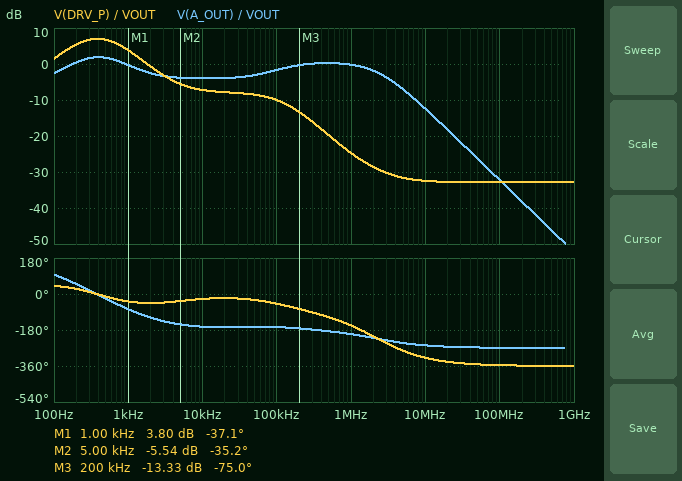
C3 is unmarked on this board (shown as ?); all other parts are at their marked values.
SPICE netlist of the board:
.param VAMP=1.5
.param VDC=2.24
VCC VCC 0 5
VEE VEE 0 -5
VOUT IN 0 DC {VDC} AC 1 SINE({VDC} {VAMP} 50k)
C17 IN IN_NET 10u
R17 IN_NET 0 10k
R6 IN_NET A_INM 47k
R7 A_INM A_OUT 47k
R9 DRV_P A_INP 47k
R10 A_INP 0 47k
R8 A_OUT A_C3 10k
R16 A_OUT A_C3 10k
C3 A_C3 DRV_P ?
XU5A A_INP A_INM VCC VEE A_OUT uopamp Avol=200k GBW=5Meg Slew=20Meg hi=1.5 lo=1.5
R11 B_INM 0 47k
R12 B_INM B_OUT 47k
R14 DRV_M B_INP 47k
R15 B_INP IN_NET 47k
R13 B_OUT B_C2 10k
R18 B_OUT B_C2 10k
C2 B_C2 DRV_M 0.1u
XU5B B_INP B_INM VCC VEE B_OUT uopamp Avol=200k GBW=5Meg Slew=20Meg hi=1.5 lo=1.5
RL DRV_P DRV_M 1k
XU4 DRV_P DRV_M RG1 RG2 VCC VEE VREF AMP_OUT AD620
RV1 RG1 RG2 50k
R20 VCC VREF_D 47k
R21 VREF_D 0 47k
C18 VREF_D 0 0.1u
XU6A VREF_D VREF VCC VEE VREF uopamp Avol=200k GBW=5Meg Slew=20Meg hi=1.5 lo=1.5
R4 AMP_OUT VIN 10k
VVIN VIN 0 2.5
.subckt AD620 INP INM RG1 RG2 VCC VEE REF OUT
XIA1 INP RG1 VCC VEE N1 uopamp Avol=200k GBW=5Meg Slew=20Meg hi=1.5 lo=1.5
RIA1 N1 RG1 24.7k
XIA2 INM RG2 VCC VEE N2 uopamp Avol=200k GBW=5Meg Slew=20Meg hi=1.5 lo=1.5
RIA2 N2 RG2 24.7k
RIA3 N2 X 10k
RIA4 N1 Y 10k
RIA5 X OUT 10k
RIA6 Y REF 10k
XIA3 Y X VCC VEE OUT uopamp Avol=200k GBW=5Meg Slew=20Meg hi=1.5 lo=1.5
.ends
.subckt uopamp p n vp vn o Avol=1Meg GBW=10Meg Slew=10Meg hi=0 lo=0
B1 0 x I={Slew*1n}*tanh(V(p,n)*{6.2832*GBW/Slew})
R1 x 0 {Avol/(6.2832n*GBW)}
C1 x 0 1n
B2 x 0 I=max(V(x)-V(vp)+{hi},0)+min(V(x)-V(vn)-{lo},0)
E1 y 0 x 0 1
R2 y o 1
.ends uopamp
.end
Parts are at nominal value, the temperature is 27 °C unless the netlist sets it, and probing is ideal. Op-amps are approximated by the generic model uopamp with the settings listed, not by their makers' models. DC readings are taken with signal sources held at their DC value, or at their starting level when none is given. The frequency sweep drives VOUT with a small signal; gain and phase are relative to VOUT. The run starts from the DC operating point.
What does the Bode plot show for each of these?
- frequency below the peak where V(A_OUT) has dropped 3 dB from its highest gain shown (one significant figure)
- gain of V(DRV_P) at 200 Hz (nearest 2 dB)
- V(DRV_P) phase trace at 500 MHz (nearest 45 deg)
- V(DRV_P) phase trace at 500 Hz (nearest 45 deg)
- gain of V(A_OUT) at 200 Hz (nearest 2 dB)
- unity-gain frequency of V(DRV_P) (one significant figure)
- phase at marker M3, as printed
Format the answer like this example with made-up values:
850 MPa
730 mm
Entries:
100 Hz
6 dB
-360 deg
0 deg
0 dB
2 kHz
-75.0 deg
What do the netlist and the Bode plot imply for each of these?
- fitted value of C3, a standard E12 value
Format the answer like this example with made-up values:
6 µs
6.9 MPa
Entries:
68 nF
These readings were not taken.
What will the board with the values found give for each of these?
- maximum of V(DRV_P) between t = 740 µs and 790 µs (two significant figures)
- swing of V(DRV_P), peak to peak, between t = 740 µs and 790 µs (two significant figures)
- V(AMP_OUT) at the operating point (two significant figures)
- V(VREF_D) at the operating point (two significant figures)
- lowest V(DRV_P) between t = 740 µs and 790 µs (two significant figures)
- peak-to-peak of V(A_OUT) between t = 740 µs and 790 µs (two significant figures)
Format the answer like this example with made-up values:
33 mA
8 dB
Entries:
560 mV
1.1 V
2.5 V
2.5 V
-570 mV
2.1 V
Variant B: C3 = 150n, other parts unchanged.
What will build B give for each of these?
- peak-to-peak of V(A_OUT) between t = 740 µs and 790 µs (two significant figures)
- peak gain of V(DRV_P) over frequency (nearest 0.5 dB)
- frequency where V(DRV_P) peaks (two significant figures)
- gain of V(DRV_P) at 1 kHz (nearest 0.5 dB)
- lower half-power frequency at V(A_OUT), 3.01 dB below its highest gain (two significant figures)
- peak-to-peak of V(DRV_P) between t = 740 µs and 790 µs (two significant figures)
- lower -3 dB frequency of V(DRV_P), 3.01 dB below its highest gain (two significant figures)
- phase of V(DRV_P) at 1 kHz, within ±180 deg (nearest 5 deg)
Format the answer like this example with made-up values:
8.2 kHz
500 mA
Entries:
2.0 V
3.0 dB
260 Hz
-2.0 dB
100 Hz
1.1 V
96 Hz
95 deg
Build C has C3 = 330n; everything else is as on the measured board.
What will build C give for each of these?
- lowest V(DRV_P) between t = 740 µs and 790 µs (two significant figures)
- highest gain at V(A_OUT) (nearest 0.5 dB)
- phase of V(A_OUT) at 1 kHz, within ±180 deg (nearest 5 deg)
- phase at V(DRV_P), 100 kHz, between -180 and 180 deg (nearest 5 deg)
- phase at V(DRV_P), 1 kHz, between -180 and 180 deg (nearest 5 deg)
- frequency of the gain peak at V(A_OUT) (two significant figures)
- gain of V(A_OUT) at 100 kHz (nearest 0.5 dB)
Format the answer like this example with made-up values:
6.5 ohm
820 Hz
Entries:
-560 mV
15.0 dB
125 deg
-45 deg
100 deg
180 Hz
-2.0 dB
